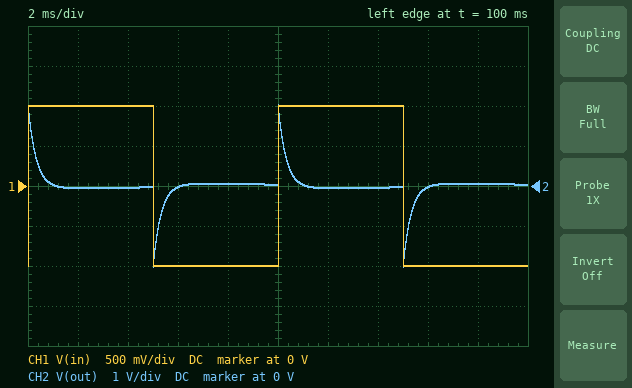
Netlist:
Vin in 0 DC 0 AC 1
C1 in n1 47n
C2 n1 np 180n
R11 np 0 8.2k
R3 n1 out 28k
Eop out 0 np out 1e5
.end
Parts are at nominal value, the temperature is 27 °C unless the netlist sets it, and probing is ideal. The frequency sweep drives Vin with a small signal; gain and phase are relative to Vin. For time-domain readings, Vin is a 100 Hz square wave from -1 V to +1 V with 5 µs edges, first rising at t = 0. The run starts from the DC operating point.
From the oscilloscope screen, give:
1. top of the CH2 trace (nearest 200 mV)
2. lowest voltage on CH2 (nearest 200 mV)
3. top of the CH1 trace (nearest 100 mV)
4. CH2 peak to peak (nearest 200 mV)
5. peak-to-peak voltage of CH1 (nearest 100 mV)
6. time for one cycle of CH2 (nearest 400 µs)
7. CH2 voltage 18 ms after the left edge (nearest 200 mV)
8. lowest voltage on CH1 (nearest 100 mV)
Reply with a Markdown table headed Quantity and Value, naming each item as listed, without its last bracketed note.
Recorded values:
| Quantity | Value |
|---|---|
| top of the CH2 trace | 2.0 V |
| lowest voltage on CH2 | -2.0 V |
| top of the CH1 trace | 1.0 V |
| CH2 peak to peak | 4.0 V |
| peak-to-peak voltage of CH1 | 2.0 V |
| time for one cycle of CH2 | 10.0 ms |
| CH2 voltage 18 ms after the left edge | 0 V |
| lowest voltage on CH1 | -1.0 V |
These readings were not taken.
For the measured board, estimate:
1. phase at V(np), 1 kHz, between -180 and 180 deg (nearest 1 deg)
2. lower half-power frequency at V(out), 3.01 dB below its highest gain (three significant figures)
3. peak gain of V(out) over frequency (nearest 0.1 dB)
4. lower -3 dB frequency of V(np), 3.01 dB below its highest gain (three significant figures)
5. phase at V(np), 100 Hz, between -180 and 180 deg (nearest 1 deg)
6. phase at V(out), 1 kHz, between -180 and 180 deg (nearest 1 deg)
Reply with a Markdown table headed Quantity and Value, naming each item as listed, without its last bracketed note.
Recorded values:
| Quantity | Value |
|---|---|
| phase at V(np), 1 kHz, between -180 and 180 deg | 28 deg |
| lower half-power frequency at V(out), 3.01 dB below its highest gain | 496 Hz |
| peak gain of V(out) over frequency | 0 dB |
| lower -3 dB frequency of V(np), 3.01 dB below its highest gain | 496 Hz |
| phase at V(np), 100 Hz, between -180 and 180 deg | 93 deg |
| phase at V(out), 1 kHz, between -180 and 180 deg | 28 deg |
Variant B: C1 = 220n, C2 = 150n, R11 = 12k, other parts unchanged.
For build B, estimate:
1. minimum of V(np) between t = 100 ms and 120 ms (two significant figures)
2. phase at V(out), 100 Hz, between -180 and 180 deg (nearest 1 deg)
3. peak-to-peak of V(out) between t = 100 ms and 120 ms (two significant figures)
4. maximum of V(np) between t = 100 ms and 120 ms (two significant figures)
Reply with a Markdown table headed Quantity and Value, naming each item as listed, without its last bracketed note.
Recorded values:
| Quantity | Value |
|---|---|
| minimum of V(np) between t = 100 ms and 120 ms | -2.1 V |
| phase at V(out), 100 Hz, between -180 and 180 deg | 63 deg |
| peak-to-peak of V(out) between t = 100 ms and 120 ms | 4.1 V |
| maximum of V(np) between t = 100 ms and 120 ms | 2.1 V |
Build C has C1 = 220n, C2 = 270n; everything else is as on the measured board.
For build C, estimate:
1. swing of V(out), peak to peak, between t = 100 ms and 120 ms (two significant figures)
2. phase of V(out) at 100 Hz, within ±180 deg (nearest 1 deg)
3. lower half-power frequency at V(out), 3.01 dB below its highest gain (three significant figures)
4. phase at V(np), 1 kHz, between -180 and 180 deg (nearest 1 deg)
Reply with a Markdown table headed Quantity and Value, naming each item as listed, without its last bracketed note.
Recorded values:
| Quantity | Value |
|---|---|
| swing of V(out), peak to peak, between t = 100 ms and 120 ms | 4.1 V |
| phase of V(out) at 100 Hz, within ±180 deg | 63 deg |
| lower half-power frequency at V(out), 3.01 dB below its highest gain | 149 Hz |
| phase at V(np), 1 kHz, between -180 and 180 deg | 9 deg |
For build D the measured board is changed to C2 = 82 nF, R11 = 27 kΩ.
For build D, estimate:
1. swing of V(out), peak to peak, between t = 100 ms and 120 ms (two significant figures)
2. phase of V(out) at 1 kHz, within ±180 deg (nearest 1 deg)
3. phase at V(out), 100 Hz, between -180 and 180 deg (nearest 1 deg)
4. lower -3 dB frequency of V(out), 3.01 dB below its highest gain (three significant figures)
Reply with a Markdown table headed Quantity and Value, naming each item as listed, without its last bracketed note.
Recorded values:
| Quantity | Value |
|---|---|
| swing of V(out), peak to peak, between t = 100 ms and 120 ms | 4.3 V |
| phase of V(out) at 1 kHz, within ±180 deg | 11 deg |
| phase at V(out), 100 Hz, between -180 and 180 deg | 86 deg |
| lower -3 dB frequency of V(out), 3.01 dB below its highest gain | 157 Hz |
